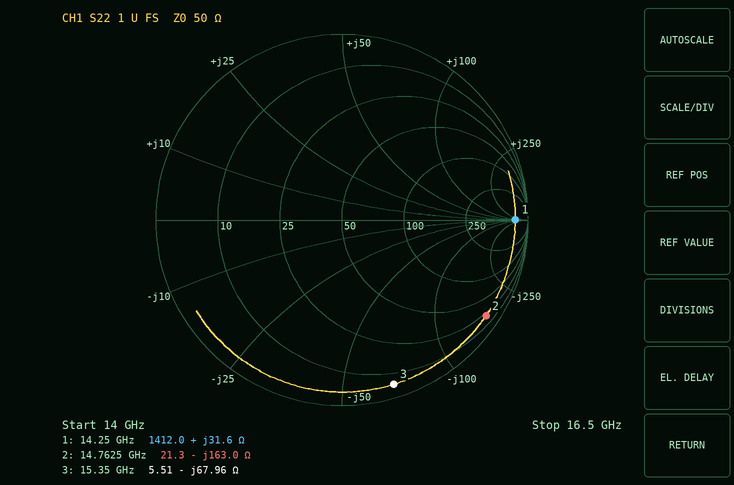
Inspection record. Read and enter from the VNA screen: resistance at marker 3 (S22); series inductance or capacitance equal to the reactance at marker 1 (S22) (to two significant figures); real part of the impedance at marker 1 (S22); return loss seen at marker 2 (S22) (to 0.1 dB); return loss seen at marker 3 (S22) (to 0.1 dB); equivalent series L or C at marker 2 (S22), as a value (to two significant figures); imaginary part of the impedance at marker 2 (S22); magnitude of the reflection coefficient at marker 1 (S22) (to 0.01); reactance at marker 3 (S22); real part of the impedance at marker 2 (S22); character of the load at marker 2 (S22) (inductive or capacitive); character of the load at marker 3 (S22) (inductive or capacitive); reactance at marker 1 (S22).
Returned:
5.51 Ω
350 pH
1412.0 Ω
0.6 dB
0.7 dB
66 fF
-163.0 Ω
0.93
-67.96 Ω
21.3 Ω
capacitive
capacitive
+31.6 Ω
